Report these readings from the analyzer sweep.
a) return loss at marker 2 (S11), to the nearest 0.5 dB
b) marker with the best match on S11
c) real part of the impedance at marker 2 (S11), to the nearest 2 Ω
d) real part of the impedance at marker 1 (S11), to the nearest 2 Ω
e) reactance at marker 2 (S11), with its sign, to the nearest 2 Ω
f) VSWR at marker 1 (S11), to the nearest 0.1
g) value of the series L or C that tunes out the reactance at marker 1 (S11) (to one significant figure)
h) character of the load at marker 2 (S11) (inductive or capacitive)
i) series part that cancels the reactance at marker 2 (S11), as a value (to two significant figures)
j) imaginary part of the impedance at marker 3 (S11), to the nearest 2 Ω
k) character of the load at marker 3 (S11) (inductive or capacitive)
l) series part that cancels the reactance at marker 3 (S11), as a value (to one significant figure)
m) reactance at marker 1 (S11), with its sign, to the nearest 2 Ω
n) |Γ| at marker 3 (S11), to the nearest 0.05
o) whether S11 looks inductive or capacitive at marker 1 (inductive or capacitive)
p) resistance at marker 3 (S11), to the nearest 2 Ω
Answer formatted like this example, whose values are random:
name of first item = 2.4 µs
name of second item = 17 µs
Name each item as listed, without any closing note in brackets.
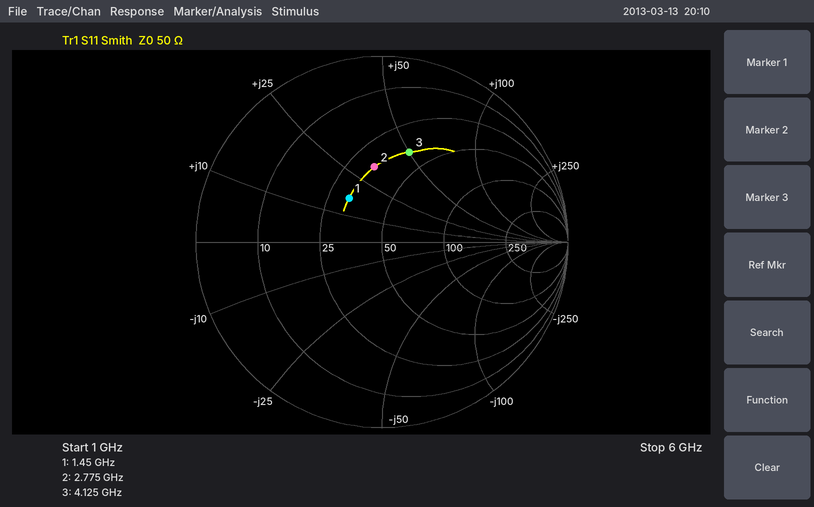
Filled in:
return loss at marker 2 (S11), to the nearest 0.5 dB = 8.0 dB
marker with the best match on S11 = marker 1
real part of the impedance at marker 2 (S11), to the nearest 2 Ω = 34 Ω
real part of the impedance at marker 1 (S11), to the nearest 2 Ω = 32 Ω
reactance at marker 2 (S11), with its sign, to the nearest 2 Ω = +32 Ω
VSWR at marker 1 (S11), to the nearest 0.1 = 1.8
value of the series L or C that tunes out the reactance at marker 1 (S11) = 7 pF
character of the load at marker 2 (S11) = inductive
series part that cancels the reactance at marker 2 (S11), as a value = 1.8 pF
imaginary part of the impedance at marker 3 (S11), to the nearest 2 Ω = +50 Ω
character of the load at marker 3 (S11) = inductive
series part that cancels the reactance at marker 3 (S11), as a value = 800 fF
reactance at marker 1 (S11), with its sign, to the nearest 2 Ω = +16 Ω
|Γ| at marker 3 (S11), to the nearest 0.05 = 0.50
whether S11 looks inductive or capacitive at marker 1 = inductive
resistance at marker 3 (S11), to the nearest 2 Ω = 38 Ω
